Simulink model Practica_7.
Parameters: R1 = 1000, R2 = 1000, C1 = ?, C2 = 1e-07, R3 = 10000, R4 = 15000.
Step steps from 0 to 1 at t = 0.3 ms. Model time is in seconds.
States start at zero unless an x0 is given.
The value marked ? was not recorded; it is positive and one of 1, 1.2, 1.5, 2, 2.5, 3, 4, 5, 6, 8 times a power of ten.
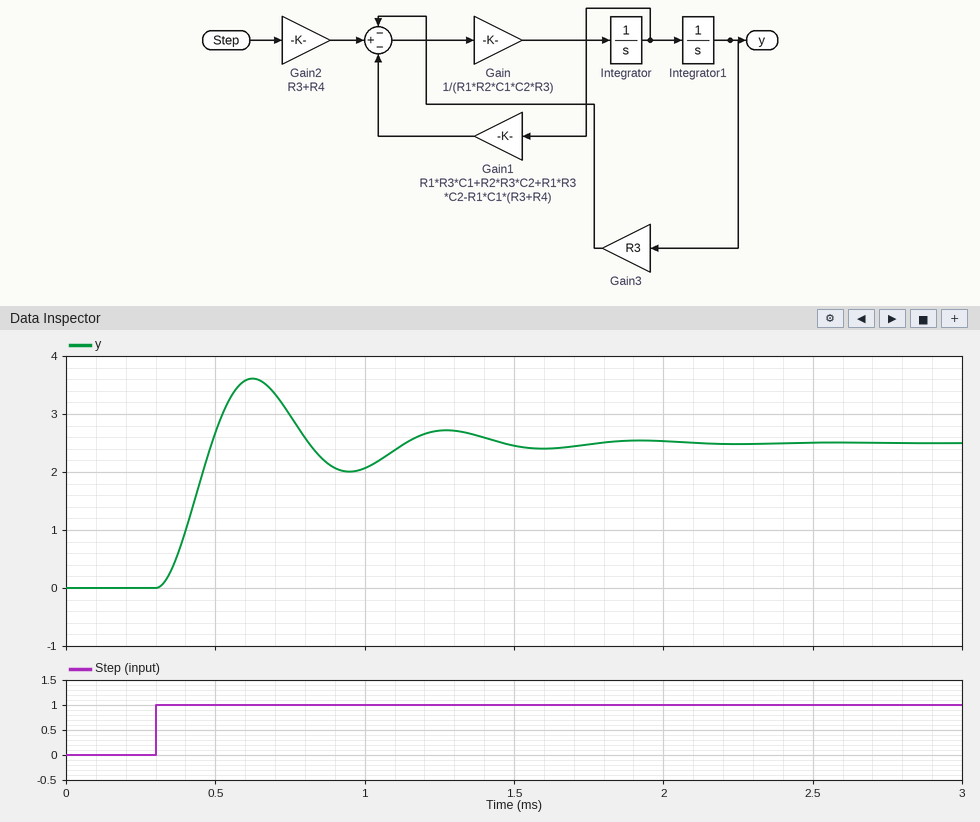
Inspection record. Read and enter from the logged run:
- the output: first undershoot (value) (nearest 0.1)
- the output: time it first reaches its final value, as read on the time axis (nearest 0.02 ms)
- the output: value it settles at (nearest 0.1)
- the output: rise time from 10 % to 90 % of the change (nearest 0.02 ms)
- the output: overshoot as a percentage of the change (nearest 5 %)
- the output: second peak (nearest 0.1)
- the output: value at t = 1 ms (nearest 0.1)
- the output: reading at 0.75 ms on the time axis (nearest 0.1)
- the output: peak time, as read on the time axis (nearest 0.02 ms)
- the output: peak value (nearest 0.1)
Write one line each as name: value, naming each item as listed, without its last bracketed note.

the output: first undershoot (value): 2.0
the output: time it first reaches its final value, as read on the time axis: 0.48 ms
the output: value it settles at: 2.5
the output: rise time from 10 % to 90 % of the change: 0.12 ms
the output: overshoot as a percentage of the change: 45 %
the output: second peak: 2.7
the output: value at t = 1 ms: 2.1
the output: reading at 0.75 ms on the time axis: 3.0
the output: peak time, as read on the time axis: 0.62 ms
the output: peak value: 3.6
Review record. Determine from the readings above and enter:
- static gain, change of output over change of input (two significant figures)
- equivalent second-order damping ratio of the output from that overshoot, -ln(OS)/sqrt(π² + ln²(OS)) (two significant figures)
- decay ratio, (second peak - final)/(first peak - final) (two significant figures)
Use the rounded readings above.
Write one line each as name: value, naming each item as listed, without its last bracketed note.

static gain, change of output over change of input: 2.5
equivalent second-order damping ratio of the output from that overshoot, -ln(OS)/sqrt(π² + ln²(OS)): 0.25
decay ratio, (second peak - final)/(first peak - final): 0.18
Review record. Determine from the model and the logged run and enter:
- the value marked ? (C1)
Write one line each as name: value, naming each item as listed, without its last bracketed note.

the value marked ?: 1e-07
